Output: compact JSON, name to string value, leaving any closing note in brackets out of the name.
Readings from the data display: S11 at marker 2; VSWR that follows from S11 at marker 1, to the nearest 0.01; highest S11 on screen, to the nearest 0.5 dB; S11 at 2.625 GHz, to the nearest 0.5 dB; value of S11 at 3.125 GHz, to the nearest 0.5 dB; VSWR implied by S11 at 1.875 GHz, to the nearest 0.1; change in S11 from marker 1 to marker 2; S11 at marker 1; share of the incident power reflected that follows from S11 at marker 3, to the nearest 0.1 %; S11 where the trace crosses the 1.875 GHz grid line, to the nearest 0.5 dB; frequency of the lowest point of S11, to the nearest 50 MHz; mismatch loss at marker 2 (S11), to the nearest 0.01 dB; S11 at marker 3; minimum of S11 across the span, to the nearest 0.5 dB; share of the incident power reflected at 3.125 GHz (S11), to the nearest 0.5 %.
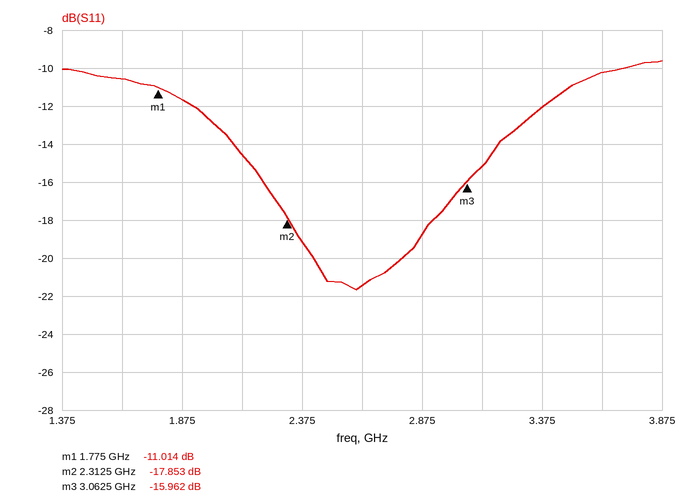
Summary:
{"S11 at marker 2": "-17.853 dB", "VSWR that follows from S11 at marker 1, to the nearest 0.01": "1.78", "highest S11 on screen, to the nearest 0.5 dB": "-9.5 dB", "S11 at 2.625 GHz, to the nearest 0.5 dB": "-21.5 dB", "value of S11 at 3.125 GHz, to the nearest 0.5 dB": "-15.0 dB", "VSWR implied by S11 at 1.875 GHz, to the nearest 0.1": "1.7", "change in S11 from marker 1 to marker 2": "-6.839 dB", "S11 at marker 1": "-11.014 dB", "share of the incident power reflected that follows from S11 at marker 3, to the nearest 0.1 %": "2.5 %", "S11 where the trace crosses the 1.875 GHz grid line, to the nearest 0.5 dB": "-11.5 dB", "frequency of the lowest point of S11, to the nearest 50 MHz": "2.60 GHz", "mismatch loss at marker 2 (S11), to the nearest 0.01 dB": "0.07 dB", "S11 at marker 3": "-15.962 dB", "minimum of S11 across the span, to the nearest 0.5 dB": "-21.5 dB", "share of the incident power reflected at 3.125 GHz (S11), to the nearest 0.5 %": "3.0 %"}
